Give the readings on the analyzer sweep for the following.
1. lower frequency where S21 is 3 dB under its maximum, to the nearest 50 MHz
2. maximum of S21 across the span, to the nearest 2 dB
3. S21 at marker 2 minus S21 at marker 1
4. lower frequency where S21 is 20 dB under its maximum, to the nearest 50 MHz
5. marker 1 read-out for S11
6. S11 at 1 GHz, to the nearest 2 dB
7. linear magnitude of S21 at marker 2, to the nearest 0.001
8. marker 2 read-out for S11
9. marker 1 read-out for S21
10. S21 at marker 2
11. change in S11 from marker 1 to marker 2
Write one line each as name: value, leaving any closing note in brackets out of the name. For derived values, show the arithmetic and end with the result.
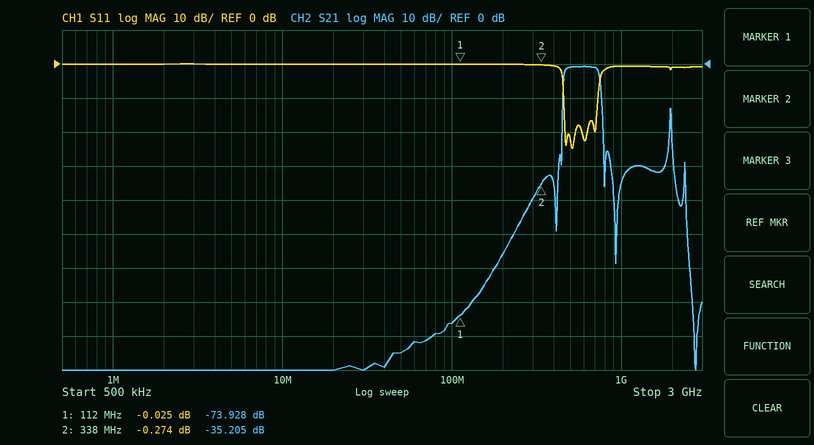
lower frequency where S21 is 3 dB under its maximum, to the nearest 50 MHz: 450 MHz
maximum of S21 across the span, to the nearest 2 dB: 0 dB
S21 at marker 2 minus S21 at marker 1: -35.205 − (-73.928) = 38.723 dB
lower frequency where S21 is 20 dB under its maximum, to the nearest 50 MHz: 450 MHz
marker 1 read-out for S11: -0.025 dB
S11 at 1 GHz, to the nearest 2 dB: 0 dB
linear magnitude of S21 at marker 2, to the nearest 0.001: 10^(-35.205/20) ≈ 0.017
marker 2 read-out for S11: -0.274 dB
marker 1 read-out for S21: -73.928 dB
S21 at marker 2: -35.205 dB
change in S11 from marker 1 to marker 2: -0.274 − (-0.025) = -0.249 dB
